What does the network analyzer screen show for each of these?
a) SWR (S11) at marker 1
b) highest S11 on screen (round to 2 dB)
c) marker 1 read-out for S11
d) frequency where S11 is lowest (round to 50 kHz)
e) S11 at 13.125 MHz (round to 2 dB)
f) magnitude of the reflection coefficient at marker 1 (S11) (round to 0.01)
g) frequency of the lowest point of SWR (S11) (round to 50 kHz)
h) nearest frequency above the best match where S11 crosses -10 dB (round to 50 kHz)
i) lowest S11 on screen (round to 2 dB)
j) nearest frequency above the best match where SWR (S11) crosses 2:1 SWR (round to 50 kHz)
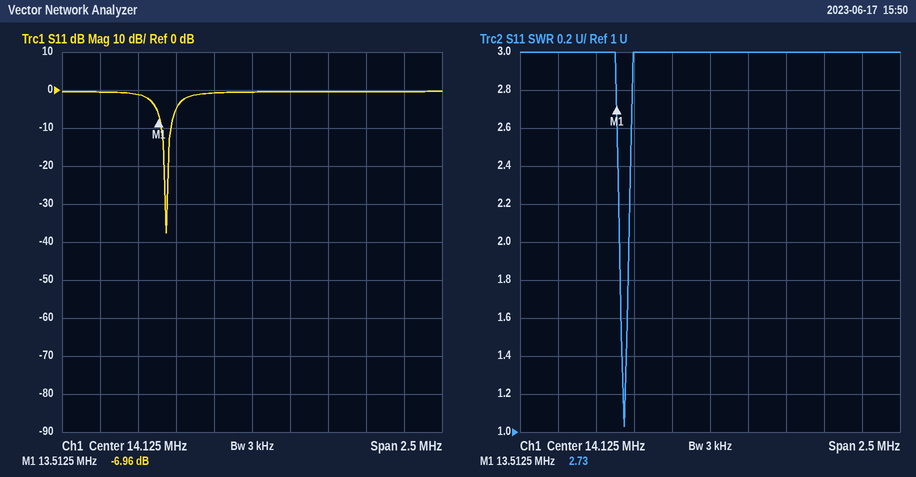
2.73
0 dB
-6.96 dB
13.55 MHz
0 dB
0.45
13.55 MHz
13.60 MHz
-38 dB
13.60 MHz
